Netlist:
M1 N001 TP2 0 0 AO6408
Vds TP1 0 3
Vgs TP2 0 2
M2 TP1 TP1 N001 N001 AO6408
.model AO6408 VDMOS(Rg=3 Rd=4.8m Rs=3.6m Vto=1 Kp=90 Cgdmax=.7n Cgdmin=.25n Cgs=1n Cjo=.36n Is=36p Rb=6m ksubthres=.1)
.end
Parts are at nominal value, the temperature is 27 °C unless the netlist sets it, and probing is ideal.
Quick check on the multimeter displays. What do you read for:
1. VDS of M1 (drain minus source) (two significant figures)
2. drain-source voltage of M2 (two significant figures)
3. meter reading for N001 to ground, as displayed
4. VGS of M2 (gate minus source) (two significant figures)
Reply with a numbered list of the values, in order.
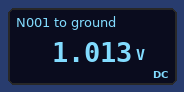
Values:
1. 1.0 V
2. 2.0 V
3. 1.013 V
4. 2.0 V
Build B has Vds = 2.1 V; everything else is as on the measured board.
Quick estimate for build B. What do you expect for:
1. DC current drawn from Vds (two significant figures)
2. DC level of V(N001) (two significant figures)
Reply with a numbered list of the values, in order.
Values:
1. 18 A
2. 400 mV
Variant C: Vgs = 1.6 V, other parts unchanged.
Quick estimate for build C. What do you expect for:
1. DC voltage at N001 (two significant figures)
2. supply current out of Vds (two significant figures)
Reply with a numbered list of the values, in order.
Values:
1. 1.4 V
2. 14 A
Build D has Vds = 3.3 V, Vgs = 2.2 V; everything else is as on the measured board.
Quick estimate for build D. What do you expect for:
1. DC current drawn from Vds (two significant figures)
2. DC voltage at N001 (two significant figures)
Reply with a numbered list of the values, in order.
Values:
1. 45 A
2. 1.1 V
